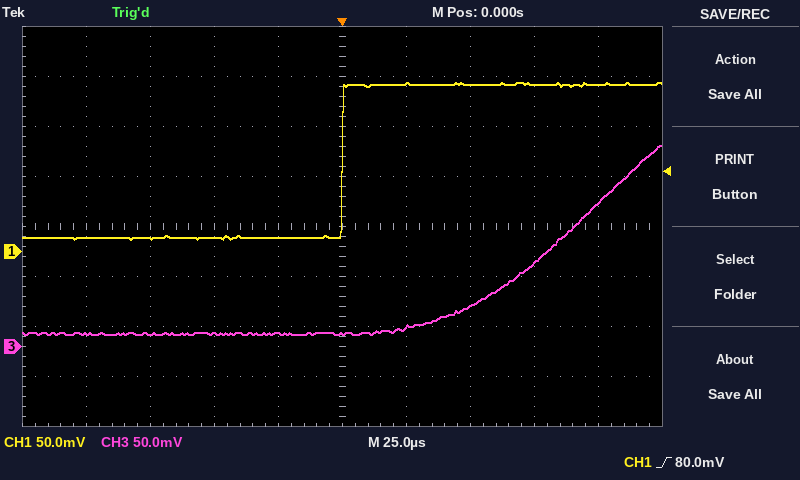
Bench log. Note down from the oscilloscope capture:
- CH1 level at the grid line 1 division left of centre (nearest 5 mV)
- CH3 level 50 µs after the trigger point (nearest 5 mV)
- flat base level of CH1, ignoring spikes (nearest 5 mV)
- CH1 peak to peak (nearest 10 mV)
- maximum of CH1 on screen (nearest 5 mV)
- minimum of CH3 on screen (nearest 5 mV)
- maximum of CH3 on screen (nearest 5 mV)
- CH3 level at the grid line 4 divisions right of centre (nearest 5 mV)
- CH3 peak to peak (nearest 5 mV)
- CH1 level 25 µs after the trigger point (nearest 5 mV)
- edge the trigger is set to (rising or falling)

15 mV
40 mV
15 mV
160 mV
170 mV
10 mV
200 mV
145 mV
190 mV
170 mV
rising
